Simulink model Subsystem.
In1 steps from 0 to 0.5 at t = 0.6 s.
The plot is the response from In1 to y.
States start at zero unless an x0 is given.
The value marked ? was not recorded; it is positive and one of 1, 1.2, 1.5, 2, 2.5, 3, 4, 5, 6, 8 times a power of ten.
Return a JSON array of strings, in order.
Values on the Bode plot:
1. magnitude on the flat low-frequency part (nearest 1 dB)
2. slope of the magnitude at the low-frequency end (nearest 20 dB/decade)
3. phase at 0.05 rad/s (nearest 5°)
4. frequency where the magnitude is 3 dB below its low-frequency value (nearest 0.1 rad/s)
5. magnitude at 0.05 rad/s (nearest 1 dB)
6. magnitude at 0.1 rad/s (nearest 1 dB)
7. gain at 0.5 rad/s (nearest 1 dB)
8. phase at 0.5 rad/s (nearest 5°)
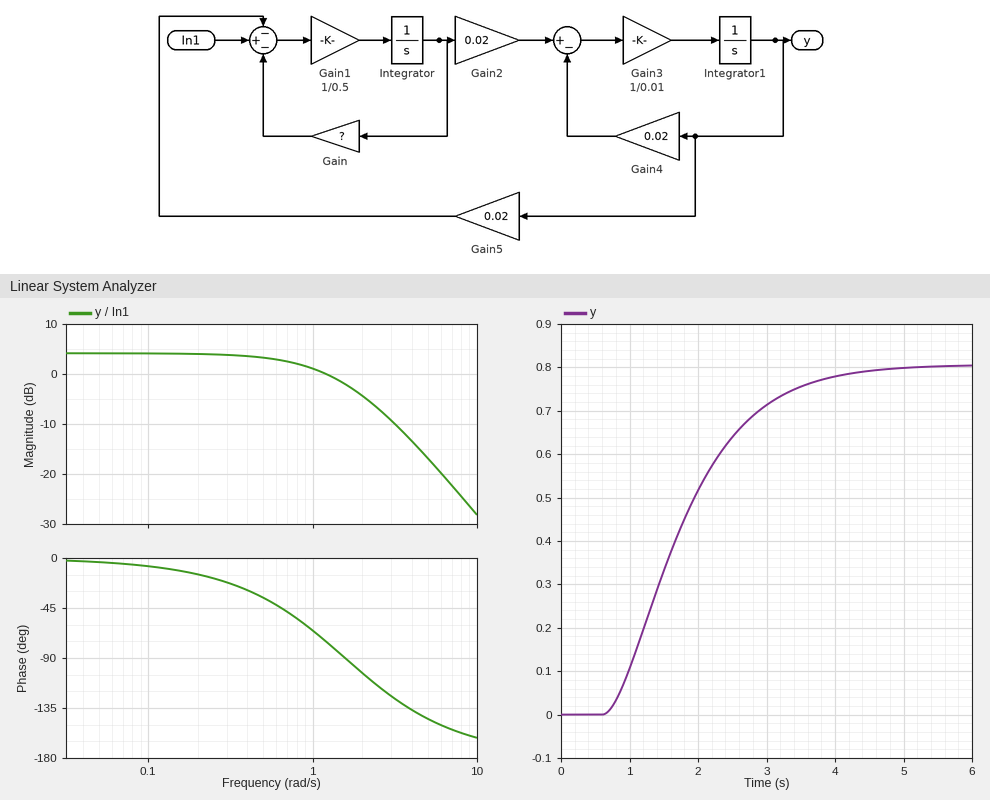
["4 dB", "0 dB/decade", "-5°", "1.0 rad/s", "4 dB", "4 dB", "3 dB", "-35°"]
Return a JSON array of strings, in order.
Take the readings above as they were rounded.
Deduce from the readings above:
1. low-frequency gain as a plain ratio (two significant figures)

["1.6"]
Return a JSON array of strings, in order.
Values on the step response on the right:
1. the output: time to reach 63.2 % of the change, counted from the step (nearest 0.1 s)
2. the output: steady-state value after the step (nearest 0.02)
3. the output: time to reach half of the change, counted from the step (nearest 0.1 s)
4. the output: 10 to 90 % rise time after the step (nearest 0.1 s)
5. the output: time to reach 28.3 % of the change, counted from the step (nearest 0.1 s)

["1.4 s", "0.80", "1.1 s", "2.2 s", "0.7 s"]
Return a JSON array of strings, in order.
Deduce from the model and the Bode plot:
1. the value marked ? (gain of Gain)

["0.6"]
